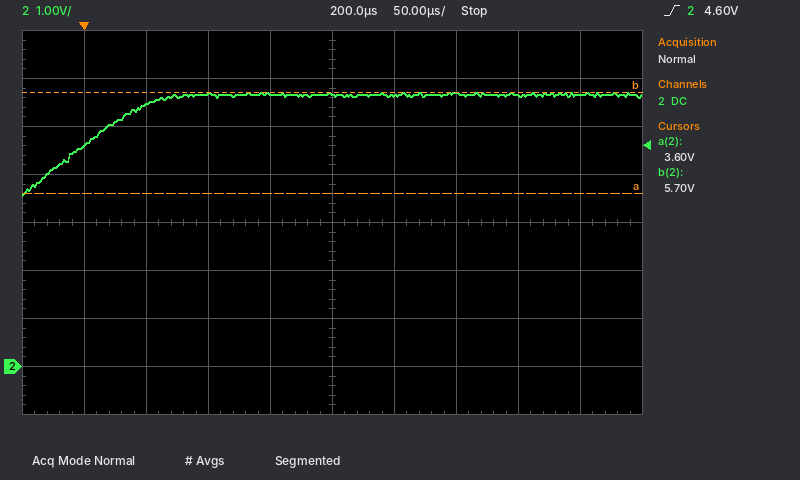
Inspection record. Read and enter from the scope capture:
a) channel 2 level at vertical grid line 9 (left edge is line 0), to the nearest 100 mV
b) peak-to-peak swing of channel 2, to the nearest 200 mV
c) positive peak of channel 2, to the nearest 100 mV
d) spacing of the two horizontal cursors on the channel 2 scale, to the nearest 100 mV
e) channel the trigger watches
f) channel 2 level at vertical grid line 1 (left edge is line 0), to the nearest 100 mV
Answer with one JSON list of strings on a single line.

["5.7 V", "2.2 V", "5.7 V", "2.1 V", "channel 2", "4.6 V"]
